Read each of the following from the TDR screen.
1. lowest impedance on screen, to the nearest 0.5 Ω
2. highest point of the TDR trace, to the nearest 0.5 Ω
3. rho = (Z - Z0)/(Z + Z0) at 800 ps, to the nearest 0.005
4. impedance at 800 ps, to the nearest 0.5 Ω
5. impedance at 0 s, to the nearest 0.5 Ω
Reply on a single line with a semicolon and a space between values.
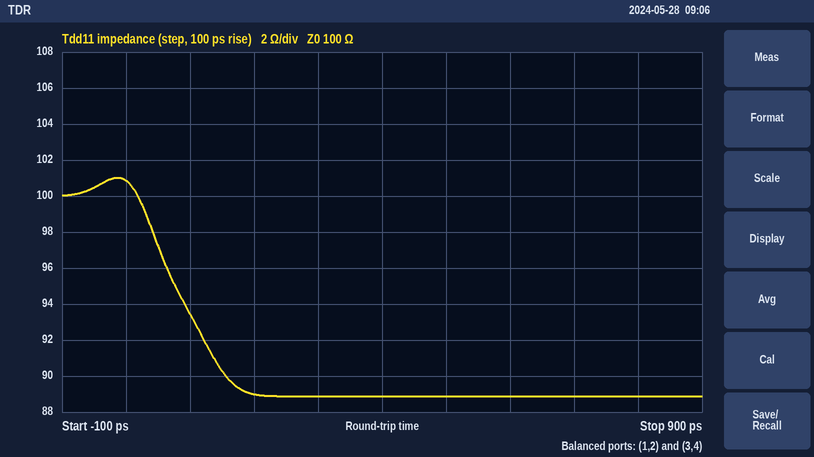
89.0 Ω; 101.0 Ω; -0.060; 89.0 Ω; 101.0 Ω
